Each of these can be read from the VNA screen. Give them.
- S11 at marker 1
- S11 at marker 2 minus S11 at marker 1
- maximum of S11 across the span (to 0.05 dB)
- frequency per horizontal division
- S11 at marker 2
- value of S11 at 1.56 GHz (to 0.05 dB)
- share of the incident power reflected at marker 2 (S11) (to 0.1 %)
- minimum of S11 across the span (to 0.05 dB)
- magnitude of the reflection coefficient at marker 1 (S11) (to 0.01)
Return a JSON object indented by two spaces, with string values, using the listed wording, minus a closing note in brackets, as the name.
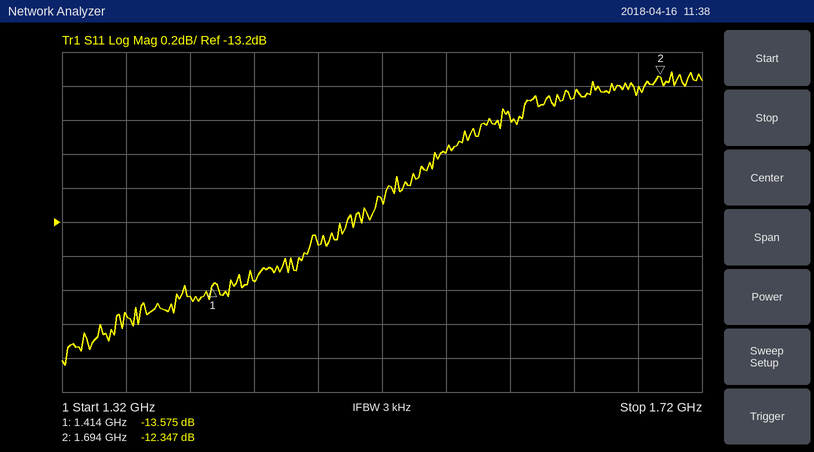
{
  "S11 at marker 1": "-13.575 dB",
  "S11 at marker 2 minus S11 at marker 1": "1.228 dB",
  "maximum of S11 across the span": "-12.30 dB",
  "frequency per horizontal division": "40 MHz",
  "S11 at marker 2": "-12.347 dB",
  "value of S11 at 1.56 GHz": "-12.80 dB",
  "share of the incident power reflected at marker 2 (S11)": "5.8 %",
  "minimum of S11 across the span": "-14.05 dB",
  "magnitude of the reflection coefficient at marker 1 (S11)": "0.21"
}
